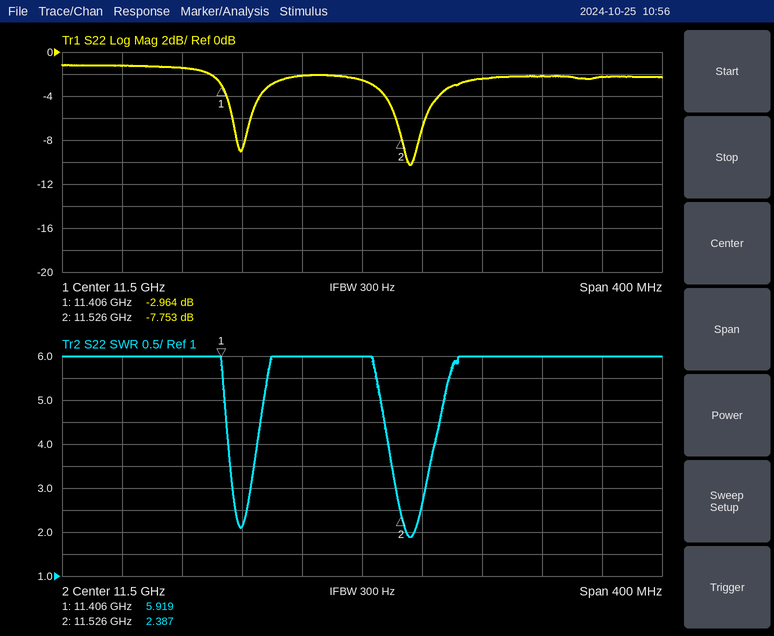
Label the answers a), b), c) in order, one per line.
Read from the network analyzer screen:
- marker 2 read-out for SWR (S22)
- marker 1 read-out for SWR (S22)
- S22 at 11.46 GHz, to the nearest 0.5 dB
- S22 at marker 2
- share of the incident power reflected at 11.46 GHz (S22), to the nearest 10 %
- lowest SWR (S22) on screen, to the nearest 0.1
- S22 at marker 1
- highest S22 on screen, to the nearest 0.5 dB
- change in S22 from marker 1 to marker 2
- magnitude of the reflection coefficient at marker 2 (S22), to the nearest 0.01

a) 2.387
b) 5.919
c) -2.0 dB
d) -7.753 dB
e) 60 %
f) 1.9
g) -2.964 dB
h) -1.0 dB
i) -4.789 dB
j) 0.41
